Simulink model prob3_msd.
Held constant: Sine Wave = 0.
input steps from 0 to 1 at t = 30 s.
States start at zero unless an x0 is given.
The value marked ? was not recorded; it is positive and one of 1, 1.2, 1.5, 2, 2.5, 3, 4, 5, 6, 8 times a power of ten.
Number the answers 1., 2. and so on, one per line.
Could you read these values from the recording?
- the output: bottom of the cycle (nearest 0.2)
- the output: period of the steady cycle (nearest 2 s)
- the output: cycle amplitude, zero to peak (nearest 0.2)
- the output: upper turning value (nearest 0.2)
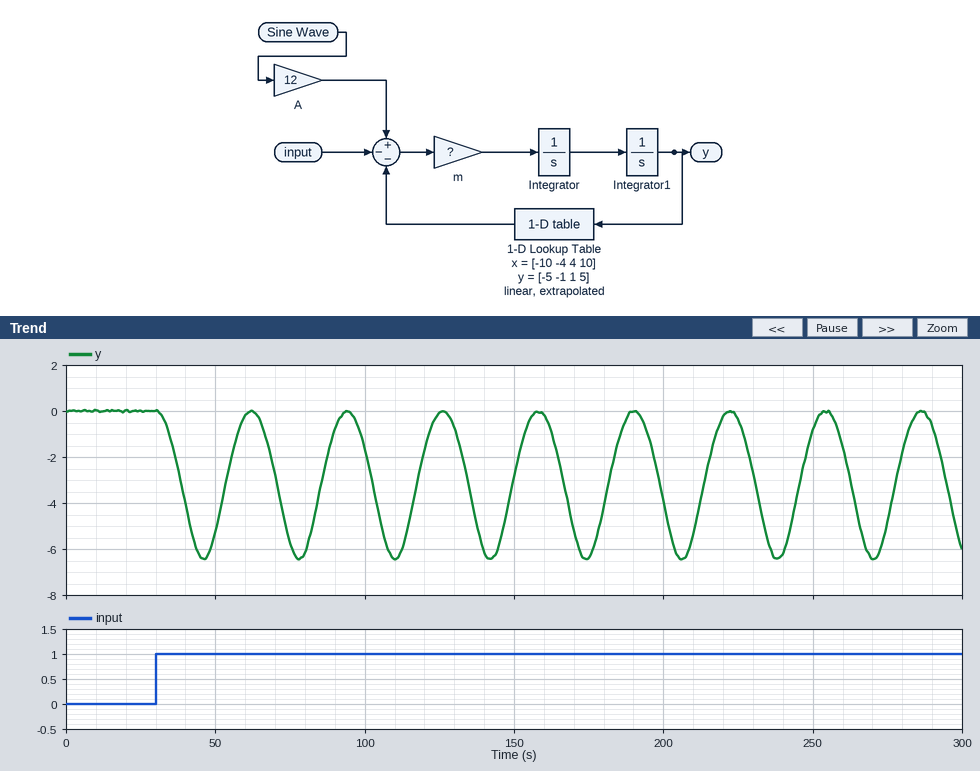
1. -6.4
2. 32 s
3. 3.2
4. 0.0
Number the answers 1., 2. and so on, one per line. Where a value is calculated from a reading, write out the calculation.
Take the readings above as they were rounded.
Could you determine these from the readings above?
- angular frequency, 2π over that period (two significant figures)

1. 2π / 32 = 0.20 rad/s
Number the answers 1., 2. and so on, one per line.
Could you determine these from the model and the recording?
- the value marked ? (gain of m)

1. 0.1
